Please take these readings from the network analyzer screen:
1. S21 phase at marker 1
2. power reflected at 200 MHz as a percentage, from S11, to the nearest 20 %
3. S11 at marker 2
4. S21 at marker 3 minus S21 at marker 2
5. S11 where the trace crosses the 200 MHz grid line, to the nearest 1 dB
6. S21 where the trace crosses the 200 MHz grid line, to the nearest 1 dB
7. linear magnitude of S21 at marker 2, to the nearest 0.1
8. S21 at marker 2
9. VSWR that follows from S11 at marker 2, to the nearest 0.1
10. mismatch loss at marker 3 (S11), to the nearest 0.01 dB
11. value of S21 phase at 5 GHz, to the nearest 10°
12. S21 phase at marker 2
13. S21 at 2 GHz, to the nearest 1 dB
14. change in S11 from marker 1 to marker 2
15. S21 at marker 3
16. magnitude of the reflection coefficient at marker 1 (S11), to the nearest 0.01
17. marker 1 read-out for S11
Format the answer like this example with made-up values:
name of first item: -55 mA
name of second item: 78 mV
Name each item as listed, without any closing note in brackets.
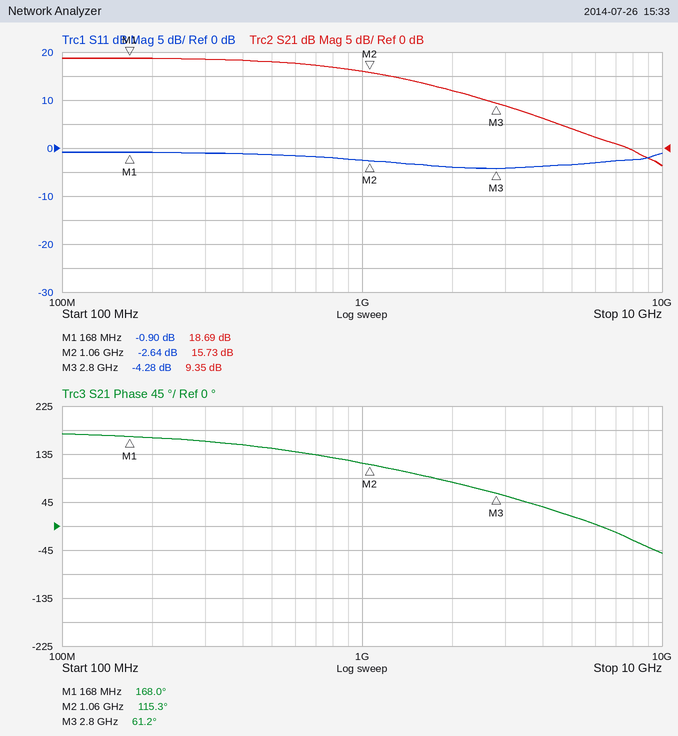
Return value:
S21 phase at marker 1: 168.0°
power reflected at 200 MHz as a percentage, from S11, to the nearest 20 %: 80 %
S11 at marker 2: -2.64 dB
S21 at marker 3 minus S21 at marker 2: -6.38 dB
S11 where the trace crosses the 200 MHz grid line, to the nearest 1 dB: -1 dB
S21 where the trace crosses the 200 MHz grid line, to the nearest 1 dB: 19 dB
linear magnitude of S21 at marker 2, to the nearest 0.1: 6.1
S21 at marker 2: 15.73 dB
VSWR that follows from S11 at marker 2, to the nearest 0.1: 6.6
mismatch loss at marker 3 (S11), to the nearest 0.01 dB: 2.03 dB
value of S21 phase at 5 GHz, to the nearest 10°: 20°
S21 phase at marker 2: 115.3°
S21 at 2 GHz, to the nearest 1 dB: 12 dB
change in S11 from marker 1 to marker 2: -1.74 dB
S21 at marker 3: 9.35 dB
magnitude of the reflection coefficient at marker 1 (S11), to the nearest 0.01: 0.90
marker 1 read-out for S11: -0.90 dB
